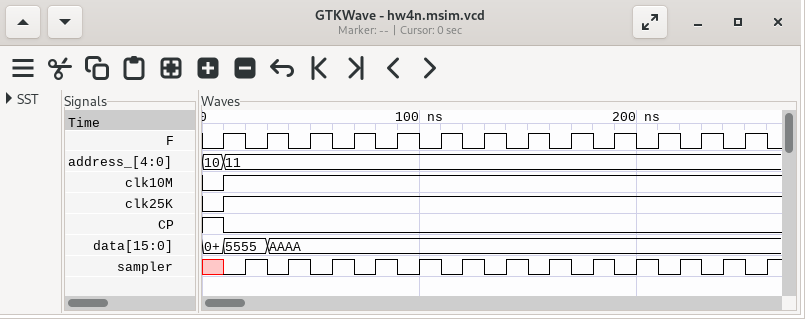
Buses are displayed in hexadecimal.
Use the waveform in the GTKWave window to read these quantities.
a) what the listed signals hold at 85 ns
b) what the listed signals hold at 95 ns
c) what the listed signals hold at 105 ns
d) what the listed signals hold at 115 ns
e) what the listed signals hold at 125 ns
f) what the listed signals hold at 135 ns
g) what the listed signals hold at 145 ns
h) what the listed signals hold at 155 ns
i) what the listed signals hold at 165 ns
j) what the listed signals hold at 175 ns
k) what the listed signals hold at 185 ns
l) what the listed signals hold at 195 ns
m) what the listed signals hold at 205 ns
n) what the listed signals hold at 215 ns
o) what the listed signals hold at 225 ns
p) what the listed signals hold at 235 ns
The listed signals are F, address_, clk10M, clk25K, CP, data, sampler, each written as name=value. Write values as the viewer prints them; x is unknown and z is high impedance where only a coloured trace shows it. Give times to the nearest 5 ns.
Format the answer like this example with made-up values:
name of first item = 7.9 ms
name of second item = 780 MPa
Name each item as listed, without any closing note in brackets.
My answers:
what the listed signals hold at 85 ns = F=0, address_=11, clk10M=1, clk25K=1, CP=0, data=AAAA, sampler=1
what the listed signals hold at 95 ns = F=1, address_=11, clk10M=1, clk25K=1, CP=0, data=AAAA, sampler=0
what the listed signals hold at 105 ns = F=0, address_=11, clk10M=1, clk25K=1, CP=0, data=AAAA, sampler=1
what the listed signals hold at 115 ns = F=1, address_=11, clk10M=1, clk25K=1, CP=0, data=AAAA, sampler=0
what the listed signals hold at 125 ns = F=0, address_=11, clk10M=1, clk25K=1, CP=0, data=AAAA, sampler=1
what the listed signals hold at 135 ns = F=1, address_=11, clk10M=1, clk25K=1, CP=0, data=AAAA, sampler=0
what the listed signals hold at 145 ns = F=0, address_=11, clk10M=1, clk25K=1, CP=0, data=AAAA, sampler=1
what the listed signals hold at 155 ns = F=1, address_=11, clk10M=1, clk25K=1, CP=0, data=AAAA, sampler=0
what the listed signals hold at 165 ns = F=0, address_=11, clk10M=1, clk25K=1, CP=0, data=AAAA, sampler=1
what the listed signals hold at 175 ns = F=1, address_=11, clk10M=1, clk25K=1, CP=0, data=AAAA, sampler=0
what the listed signals hold at 185 ns = F=0, address_=11, clk10M=1, clk25K=1, CP=0, data=AAAA, sampler=1
what the listed signals hold at 195 ns = F=1, address_=11, clk10M=1, clk25K=1, CP=0, data=AAAA, sampler=0
what the listed signals hold at 205 ns = F=0, address_=11, clk10M=1, clk25K=1, CP=0, data=AAAA, sampler=1
what the listed signals hold at 215 ns = F=1, address_=11, clk10M=1, clk25K=1, CP=0, data=AAAA, sampler=0
what the listed signals hold at 225 ns = F=0, address_=11, clk10M=1, clk25K=1, CP=0, data=AAAA, sampler=1
what the listed signals hold at 235 ns = F=1, address_=11, clk10M=1, clk25K=1, CP=0, data=AAAA, sampler=0
